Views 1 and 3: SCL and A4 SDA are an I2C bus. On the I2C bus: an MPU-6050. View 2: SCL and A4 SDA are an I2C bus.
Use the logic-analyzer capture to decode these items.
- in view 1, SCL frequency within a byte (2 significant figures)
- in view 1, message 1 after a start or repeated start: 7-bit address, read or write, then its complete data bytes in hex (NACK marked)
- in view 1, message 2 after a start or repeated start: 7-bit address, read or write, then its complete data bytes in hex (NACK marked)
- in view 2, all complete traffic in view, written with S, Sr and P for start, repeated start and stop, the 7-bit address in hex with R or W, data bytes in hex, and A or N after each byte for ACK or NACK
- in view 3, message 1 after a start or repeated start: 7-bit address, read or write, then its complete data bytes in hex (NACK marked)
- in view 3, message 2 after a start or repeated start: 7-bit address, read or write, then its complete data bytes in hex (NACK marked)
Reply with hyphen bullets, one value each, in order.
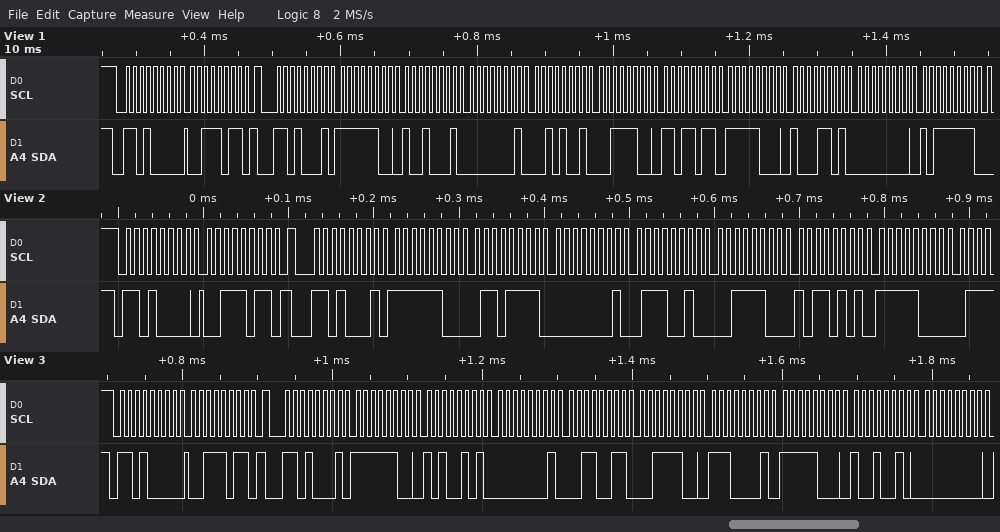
- 100 kHz
- 0x68 write: 3B
- 0x68 read: FC 91 01 29 3C DB F8 8D 00 BF
- S 68W A 3B A Sr 68R A FC A 6F A 01 A 72 A 3C A B5 A F8 A
- 0x68 write: 3B
- 0x68 read: FC A5 01 33 3C E1 F8 92 00
